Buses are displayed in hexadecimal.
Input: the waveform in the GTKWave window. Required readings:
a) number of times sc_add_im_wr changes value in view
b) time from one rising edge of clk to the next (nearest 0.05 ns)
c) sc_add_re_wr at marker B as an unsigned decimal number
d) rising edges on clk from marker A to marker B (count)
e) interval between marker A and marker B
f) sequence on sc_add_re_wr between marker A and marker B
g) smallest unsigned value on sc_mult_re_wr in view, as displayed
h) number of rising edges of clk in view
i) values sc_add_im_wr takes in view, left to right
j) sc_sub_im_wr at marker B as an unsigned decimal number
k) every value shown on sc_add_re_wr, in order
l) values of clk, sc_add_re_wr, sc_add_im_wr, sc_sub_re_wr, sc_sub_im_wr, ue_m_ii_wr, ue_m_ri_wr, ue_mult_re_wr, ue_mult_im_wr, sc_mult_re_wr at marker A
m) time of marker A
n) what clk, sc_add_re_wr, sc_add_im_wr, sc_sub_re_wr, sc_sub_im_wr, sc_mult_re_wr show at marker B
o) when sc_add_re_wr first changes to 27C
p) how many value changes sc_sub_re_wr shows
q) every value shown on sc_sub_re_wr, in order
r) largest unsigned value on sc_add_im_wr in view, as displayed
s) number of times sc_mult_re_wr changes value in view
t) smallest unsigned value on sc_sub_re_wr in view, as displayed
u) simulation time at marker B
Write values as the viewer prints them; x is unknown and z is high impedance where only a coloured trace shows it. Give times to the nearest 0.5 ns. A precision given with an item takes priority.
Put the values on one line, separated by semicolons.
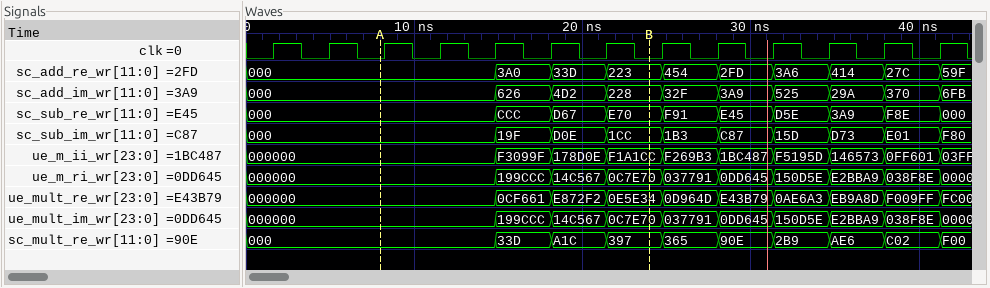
9; 3.3 ns; 547; 5; 16 ns; 000, 3A0, 33D, 223; 000; 13; 000, 626, 4D2, 228, 32F, 3A9, 525, 29A, 370, 6FB; 460; 000, 3A0, 33D, 223, 454, 2FD, 3A6, 414, 27C, 59F; clk=0, sc_add_re_wr=000, sc_add_im_wr=000, sc_sub_re_wr=000, sc_sub_im_wr=000, ue_m_ii_wr=000000, ue_m_ri_wr=000000, ue_mult_re_wr=000000, ue_mult_im_wr=000000, sc_mult_re_wr=000; 8 ns; clk=0, sc_add_re_wr=223, sc_add_im_wr=228, sc_sub_re_wr=E70, sc_sub_im_wr=1CC, sc_mult_re_wr=397; 38 ns; 9; 000, CCC, D67, E70, F91, E45, D5E, 3A9, F8E, 000; 6FB; 9; 000; 24 ns
